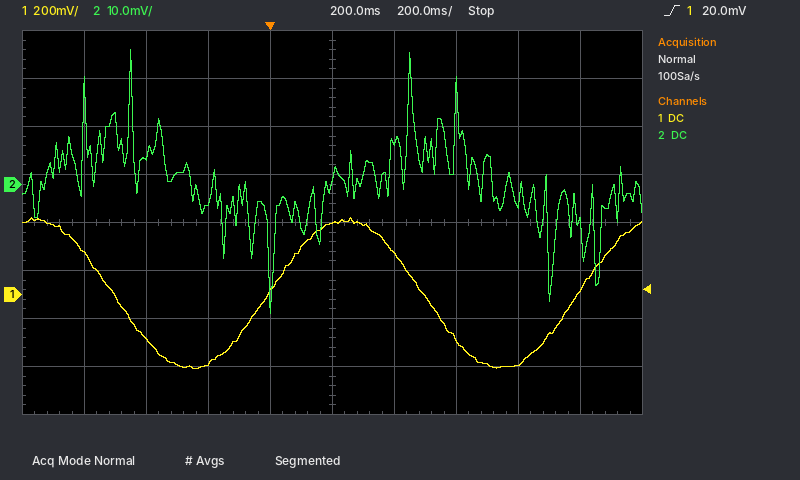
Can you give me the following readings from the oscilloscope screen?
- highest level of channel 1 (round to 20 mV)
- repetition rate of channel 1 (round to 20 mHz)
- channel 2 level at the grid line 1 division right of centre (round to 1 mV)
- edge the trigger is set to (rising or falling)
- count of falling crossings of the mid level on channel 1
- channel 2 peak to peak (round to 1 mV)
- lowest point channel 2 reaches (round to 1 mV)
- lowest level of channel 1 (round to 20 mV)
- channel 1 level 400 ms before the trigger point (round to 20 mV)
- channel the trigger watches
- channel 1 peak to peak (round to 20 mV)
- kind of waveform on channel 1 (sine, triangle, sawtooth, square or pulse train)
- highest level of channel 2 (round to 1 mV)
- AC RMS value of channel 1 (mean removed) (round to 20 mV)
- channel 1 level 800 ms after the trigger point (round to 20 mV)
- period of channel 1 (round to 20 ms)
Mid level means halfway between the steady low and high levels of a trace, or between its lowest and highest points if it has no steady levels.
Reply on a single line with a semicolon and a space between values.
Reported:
320 mV; 1.00 Hz; 9 mV; rising; 2; 55 mV; -27 mV; -300 mV; -180 mV; channel 1; 620 mV; sine; 28 mV; 220 mV; -300 mV; 1.00 s
